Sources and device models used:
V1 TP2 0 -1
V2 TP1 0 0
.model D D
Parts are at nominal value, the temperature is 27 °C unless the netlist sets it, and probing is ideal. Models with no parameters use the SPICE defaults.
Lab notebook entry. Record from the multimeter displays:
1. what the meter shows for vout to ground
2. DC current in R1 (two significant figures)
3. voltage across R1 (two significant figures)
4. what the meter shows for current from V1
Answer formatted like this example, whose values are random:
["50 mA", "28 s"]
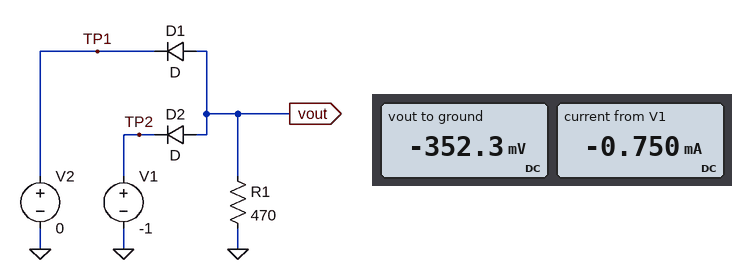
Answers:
["-352.3 mV", "750 µA", "350 mV", "-0.750 mA"]
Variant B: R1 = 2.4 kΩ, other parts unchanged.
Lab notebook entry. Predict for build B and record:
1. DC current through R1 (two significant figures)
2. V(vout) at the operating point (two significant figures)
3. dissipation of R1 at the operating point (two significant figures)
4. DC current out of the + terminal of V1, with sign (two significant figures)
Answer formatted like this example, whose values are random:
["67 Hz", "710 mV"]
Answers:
["160 µA", "-390 mV", "64 µW", "-160 µA"]
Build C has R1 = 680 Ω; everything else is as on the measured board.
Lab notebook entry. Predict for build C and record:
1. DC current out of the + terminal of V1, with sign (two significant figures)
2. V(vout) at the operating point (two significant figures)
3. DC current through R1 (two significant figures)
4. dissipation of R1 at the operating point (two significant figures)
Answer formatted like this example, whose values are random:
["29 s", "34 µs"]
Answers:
["-530 µA", "-360 mV", "530 µA", "190 µW"]
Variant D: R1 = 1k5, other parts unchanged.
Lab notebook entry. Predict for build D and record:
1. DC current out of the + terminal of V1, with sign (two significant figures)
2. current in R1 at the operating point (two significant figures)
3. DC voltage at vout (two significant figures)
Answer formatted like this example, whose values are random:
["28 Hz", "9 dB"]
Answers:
["-250 µA", "250 µA", "-380 mV"]
